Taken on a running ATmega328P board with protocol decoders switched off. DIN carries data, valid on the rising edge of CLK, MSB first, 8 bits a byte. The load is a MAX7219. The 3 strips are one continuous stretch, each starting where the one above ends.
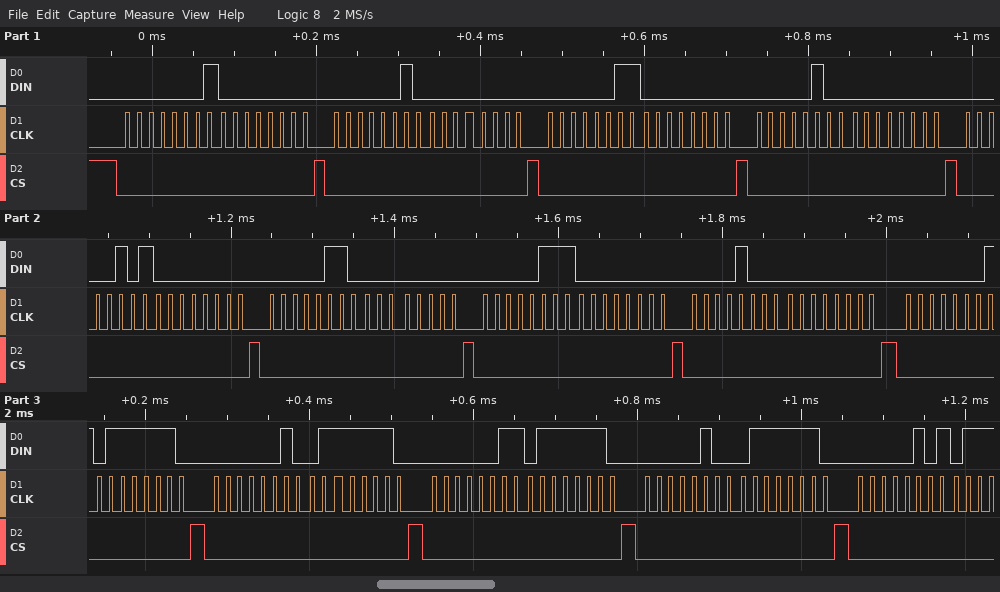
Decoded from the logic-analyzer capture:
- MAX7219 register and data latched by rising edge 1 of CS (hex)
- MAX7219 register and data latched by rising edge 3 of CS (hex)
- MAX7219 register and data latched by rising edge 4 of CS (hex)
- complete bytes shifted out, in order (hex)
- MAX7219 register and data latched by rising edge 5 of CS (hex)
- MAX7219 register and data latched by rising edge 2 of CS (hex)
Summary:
register 0x1, data 0x00
register 0x3, data 0x00
register 0x4, data 0x00
01 00 02 00 03 00 04 00 05 00 06 00 07 00 08 00 01 7E 02 7E 03 7E 04 7E 05
register 0x5, data 0x00
register 0x2, data 0x00
